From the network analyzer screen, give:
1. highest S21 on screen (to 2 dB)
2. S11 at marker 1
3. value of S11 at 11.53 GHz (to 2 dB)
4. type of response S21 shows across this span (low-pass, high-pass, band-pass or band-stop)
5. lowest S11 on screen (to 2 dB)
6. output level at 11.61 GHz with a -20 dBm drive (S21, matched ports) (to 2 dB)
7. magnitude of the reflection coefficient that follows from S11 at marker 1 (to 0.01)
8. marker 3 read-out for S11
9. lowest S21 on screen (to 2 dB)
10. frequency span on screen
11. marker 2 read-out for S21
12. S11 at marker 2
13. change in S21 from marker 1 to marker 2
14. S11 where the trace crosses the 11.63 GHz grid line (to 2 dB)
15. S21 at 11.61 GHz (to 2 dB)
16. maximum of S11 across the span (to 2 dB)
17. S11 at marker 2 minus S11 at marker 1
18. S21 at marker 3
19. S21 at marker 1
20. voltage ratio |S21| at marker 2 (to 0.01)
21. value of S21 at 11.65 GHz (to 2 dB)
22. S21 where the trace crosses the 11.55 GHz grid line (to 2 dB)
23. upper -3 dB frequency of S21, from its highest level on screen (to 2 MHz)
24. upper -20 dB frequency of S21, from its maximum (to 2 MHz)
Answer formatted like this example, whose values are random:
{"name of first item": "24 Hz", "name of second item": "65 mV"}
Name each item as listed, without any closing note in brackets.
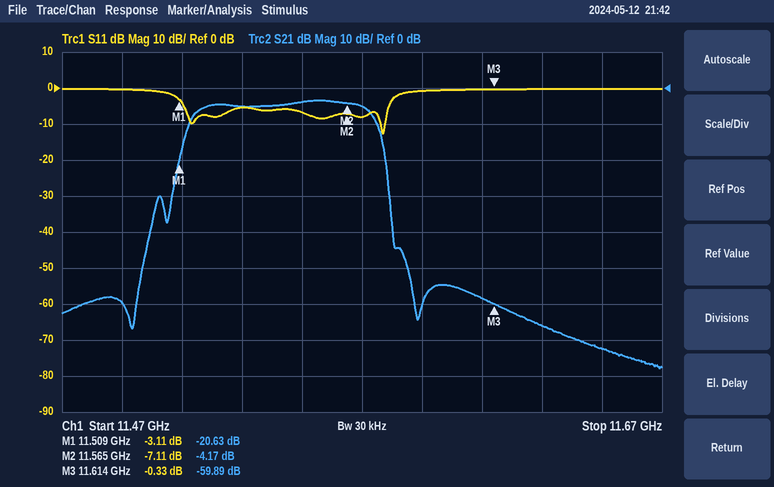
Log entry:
{"highest S21 on screen": "-4 dB", "S11 at marker 1": "-3.11 dB", "value of S11 at 11.53 GHz": "-6 dB", "type of response S21 shows across this span": "band-pass", "lowest S11 on screen": "-12 dB", "output level at 11.61 GHz with a -20 dBm drive (S21, matched ports)": "-78 dBm", "magnitude of the reflection coefficient that follows from S11 at marker 1": "0.70", "marker 3 read-out for S11": "-0.33 dB", "lowest S21 on screen": "-78 dB", "frequency span on screen": "200 MHz", "marker 2 read-out for S21": "-4.17 dB", "S11 at marker 2": "-7.11 dB", "change in S21 from marker 1 to marker 2": "16.46 dB", "S11 where the trace crosses the 11.63 GHz grid line": "0 dB", "S21 at 11.61 GHz": "-58 dB", "maximum of S11 across the span": "0 dB", "S11 at marker 2 minus S11 at marker 1": "-4.00 dB", "S21 at marker 3": "-59.89 dB", "S21 at marker 1": "-20.63 dB", "voltage ratio |S21| at marker 2": "0.62", "value of S21 at 11.65 GHz": "-72 dB", "S21 where the trace crosses the 11.55 GHz grid line": "-4 dB", "upper -3 dB frequency of S21, from its highest level on screen": "11.572 GHz", "upper -20 dB frequency of S21, from its maximum": "11.578 GHz"}
